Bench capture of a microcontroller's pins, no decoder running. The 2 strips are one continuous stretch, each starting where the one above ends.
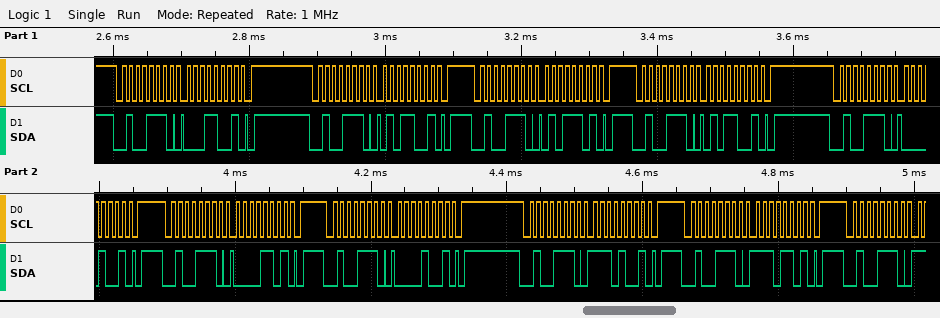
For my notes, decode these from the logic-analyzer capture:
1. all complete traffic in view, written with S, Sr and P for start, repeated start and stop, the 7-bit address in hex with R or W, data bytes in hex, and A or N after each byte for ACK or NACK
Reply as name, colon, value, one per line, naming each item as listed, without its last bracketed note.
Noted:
all complete traffic in view, written with S, Sr and P for start, repeated start and stop, the 7-bit address in hex with R or W, data bytes in hex, and A or N after each byte for ACK or NACK: S 27W A 19 A P S 27W A 59 A P S 27W A 5D A P S 27W A 59 A P S 27W A 09 A P S 27W A 0D A P S 27W A 09 A P S 27W A E9 A P S 27W A ED A P S 27W A
